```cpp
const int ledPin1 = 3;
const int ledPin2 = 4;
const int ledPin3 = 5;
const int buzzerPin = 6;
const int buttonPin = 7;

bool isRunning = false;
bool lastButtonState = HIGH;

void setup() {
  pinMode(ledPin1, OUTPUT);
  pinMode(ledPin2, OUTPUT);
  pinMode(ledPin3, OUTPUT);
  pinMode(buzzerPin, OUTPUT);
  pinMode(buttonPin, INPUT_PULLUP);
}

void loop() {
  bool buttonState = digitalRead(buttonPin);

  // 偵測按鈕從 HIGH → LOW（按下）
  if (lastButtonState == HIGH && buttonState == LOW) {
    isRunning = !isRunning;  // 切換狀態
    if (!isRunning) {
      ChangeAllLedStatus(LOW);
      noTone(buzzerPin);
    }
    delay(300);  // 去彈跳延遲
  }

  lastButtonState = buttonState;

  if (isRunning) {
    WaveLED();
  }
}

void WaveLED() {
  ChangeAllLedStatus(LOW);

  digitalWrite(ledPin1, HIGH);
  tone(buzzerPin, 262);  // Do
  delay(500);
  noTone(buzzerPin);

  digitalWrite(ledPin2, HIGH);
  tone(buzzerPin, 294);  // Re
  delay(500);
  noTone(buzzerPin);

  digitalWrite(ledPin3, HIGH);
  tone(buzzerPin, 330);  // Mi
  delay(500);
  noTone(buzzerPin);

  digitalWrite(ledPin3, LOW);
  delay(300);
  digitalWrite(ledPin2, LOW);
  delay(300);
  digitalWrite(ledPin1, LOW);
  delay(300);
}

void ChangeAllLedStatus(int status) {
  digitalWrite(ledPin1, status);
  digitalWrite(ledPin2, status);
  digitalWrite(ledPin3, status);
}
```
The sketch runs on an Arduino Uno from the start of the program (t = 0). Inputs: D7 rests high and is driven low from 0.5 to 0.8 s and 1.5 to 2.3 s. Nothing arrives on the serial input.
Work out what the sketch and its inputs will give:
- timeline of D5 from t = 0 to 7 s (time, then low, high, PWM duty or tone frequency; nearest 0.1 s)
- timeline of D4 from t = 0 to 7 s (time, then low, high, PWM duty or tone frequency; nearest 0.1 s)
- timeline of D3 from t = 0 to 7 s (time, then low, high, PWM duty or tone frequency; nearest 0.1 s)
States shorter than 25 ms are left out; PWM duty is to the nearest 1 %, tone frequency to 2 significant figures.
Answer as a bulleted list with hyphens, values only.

- 0 s low; 1.8 s high; 2.3 s low; 4.2 s high; 4.7 s low; 6.6 s high
- 0 s low; 1.3 s high; 2.6 s low; 3.7 s high; 5 s low; 6.1 s high
- 0 s low; 0.8 s high; 2.9 s low; 3.2 s high; 5.3 s low; 5.6 s high
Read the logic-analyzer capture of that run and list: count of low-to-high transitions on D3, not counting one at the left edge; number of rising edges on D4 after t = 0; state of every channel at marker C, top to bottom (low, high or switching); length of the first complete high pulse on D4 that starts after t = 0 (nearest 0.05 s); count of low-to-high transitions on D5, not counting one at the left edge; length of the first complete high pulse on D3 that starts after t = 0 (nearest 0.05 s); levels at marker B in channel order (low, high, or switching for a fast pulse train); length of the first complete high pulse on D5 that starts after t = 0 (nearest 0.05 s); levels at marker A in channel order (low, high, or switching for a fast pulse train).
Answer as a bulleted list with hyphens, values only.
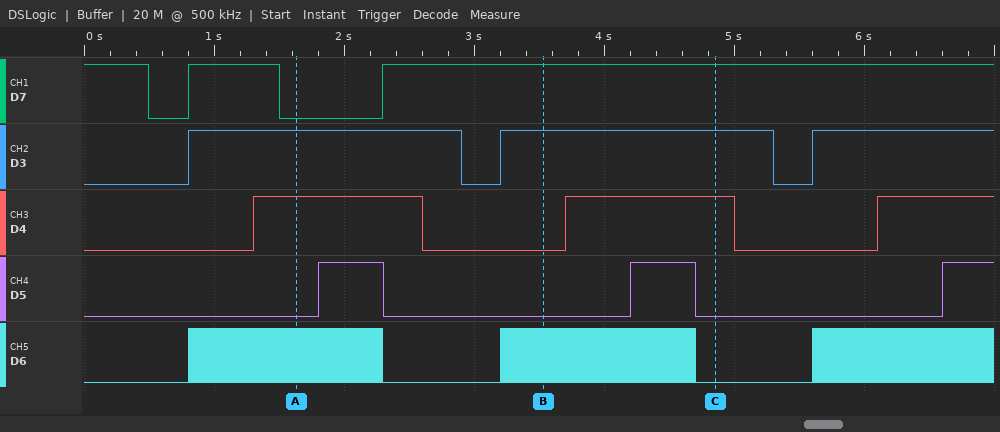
- 3
- 3
- D7 high, D3 high, D4 high, D5 low, D6 low
- 1.30 s
- 3
- 2.10 s
- D7 high, D3 high, D4 low, D5 low, D6 switching
- 0.50 s
- D7 low, D3 high, D4 high, D5 low, D6 switching
